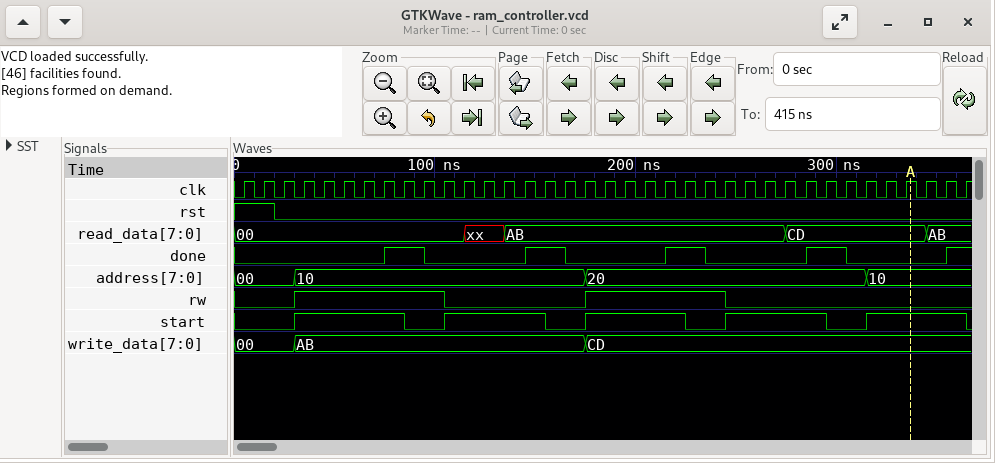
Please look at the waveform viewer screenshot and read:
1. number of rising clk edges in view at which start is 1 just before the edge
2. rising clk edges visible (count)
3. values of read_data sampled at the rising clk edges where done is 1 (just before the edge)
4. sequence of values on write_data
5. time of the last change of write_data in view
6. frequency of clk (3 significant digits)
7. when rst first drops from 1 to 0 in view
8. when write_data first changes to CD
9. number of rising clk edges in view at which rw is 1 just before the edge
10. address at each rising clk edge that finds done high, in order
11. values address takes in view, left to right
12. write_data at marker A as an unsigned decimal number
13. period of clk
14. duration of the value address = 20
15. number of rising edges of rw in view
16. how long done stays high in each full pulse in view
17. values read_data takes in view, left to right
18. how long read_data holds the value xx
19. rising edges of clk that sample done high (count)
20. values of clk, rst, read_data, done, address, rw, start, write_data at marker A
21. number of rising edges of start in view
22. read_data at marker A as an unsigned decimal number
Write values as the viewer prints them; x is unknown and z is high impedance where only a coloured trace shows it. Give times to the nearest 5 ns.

26
37
00, 00, AB, AB, AB, AB, CD, CD, AB
00, AB, CD
175 ns
100 MHz
20 ns
175 ns
15
10, 10, 10, 10, 20, 20, 20, 20, 10
00, 10, 20, 10
205
10 ns
140 ns
2
20 ns, 20 ns, 20 ns, 20 ns
00, xx, AB, CD, AB
20 ns
9
clk=1, rst=0, read_data=CD, done=0, address=10, rw=0, start=1, write_data=CD
5
205
